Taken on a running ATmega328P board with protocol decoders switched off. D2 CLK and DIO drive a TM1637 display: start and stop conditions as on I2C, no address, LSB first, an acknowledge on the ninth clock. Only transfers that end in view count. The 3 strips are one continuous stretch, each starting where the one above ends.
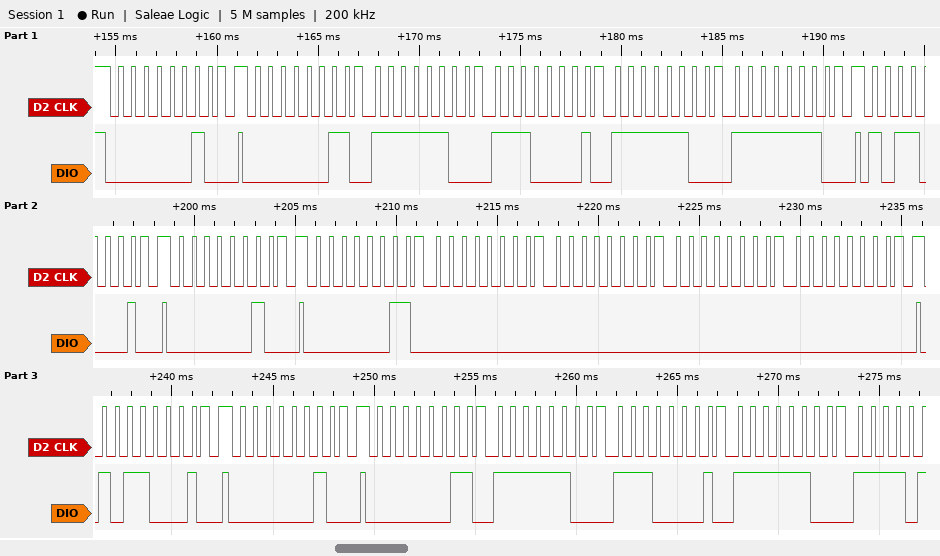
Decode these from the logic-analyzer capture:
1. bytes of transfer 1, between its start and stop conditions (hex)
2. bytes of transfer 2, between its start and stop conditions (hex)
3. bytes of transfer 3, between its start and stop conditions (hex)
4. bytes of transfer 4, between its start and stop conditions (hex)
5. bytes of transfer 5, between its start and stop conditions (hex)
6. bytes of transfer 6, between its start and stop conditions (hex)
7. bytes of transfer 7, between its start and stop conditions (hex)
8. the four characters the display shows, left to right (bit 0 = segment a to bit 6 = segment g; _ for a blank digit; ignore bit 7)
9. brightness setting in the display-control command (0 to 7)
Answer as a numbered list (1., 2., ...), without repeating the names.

1. 40
2. C0 3F 87 3F 7F
3. 8D
4. 40
5. C0 00 00 00 00
6. 8D
7. 40
8. ____
9. 5
